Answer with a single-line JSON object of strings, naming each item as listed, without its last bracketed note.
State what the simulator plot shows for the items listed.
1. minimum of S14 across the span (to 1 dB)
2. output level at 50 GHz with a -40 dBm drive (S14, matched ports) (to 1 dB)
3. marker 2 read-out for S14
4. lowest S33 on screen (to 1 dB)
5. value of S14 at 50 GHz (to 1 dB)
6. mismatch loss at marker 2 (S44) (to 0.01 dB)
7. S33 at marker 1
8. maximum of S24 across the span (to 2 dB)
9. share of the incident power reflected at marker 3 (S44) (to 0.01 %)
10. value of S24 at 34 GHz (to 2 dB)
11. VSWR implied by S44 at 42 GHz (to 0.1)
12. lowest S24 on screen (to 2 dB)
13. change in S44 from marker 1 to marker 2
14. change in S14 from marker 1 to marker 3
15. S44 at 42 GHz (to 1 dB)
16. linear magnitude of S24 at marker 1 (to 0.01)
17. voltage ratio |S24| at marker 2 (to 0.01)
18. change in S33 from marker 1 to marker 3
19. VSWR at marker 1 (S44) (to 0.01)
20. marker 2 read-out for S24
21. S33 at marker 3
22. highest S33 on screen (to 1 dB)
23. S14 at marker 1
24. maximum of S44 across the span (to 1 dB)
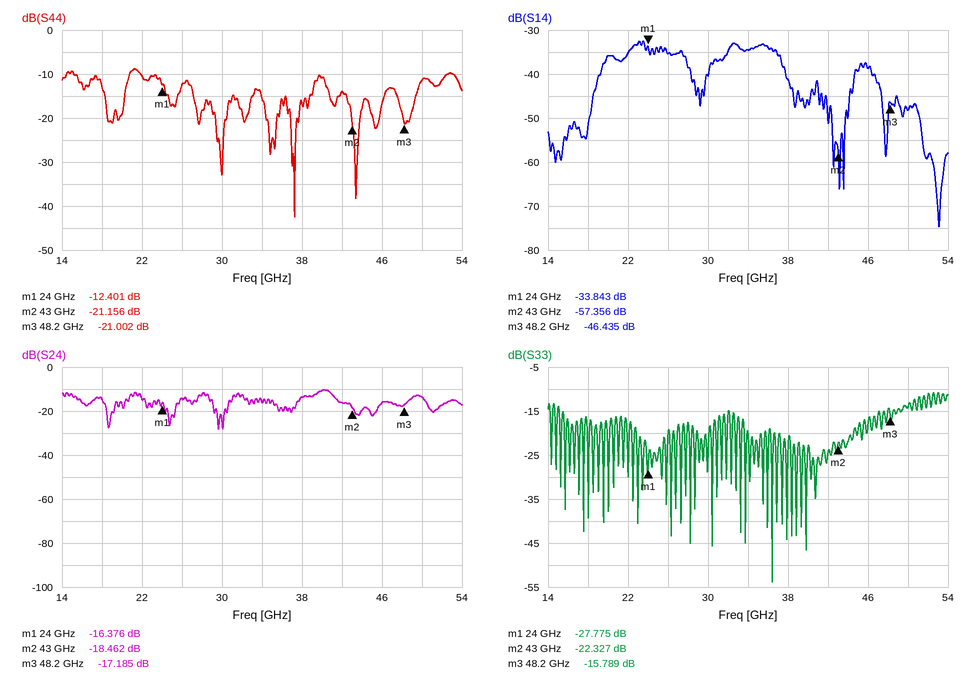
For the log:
{"minimum of S14 across the span": "-75 dB", "output level at 50 GHz with a -40 dBm drive (S14, matched ports)": "-88 dBm", "marker 2 read-out for S14": "-57.356 dB", "lowest S33 on screen": "-54 dB", "value of S14 at 50 GHz": "-48 dB", "mismatch loss at marker 2 (S44)": "0.03 dB", "S33 at marker 1": "-27.775 dB", "maximum of S24 across the span": "-10 dB", "share of the incident power reflected at marker 3 (S44)": "0.79 %", "value of S24 at 34 GHz": "-16 dB", "VSWR implied by S44 at 42 GHz": "1.5", "lowest S24 on screen": "-28 dB", "change in S44 from marker 1 to marker 2": "-8.755 dB", "change in S14 from marker 1 to marker 3": "-12.592 dB", "S44 at 42 GHz": "-14 dB", "linear magnitude of S24 at marker 1": "0.15", "voltage ratio |S24| at marker 2": "0.12", "change in S33 from marker 1 to marker 3": "11.986 dB", "VSWR at marker 1 (S44)": "1.63", "marker 2 read-out for S24": "-18.462 dB", "S33 at marker 3": "-15.789 dB", "highest S33 on screen": "-11 dB", "S14 at marker 1": "-33.843 dB", "maximum of S44 across the span": "-9 dB"}
